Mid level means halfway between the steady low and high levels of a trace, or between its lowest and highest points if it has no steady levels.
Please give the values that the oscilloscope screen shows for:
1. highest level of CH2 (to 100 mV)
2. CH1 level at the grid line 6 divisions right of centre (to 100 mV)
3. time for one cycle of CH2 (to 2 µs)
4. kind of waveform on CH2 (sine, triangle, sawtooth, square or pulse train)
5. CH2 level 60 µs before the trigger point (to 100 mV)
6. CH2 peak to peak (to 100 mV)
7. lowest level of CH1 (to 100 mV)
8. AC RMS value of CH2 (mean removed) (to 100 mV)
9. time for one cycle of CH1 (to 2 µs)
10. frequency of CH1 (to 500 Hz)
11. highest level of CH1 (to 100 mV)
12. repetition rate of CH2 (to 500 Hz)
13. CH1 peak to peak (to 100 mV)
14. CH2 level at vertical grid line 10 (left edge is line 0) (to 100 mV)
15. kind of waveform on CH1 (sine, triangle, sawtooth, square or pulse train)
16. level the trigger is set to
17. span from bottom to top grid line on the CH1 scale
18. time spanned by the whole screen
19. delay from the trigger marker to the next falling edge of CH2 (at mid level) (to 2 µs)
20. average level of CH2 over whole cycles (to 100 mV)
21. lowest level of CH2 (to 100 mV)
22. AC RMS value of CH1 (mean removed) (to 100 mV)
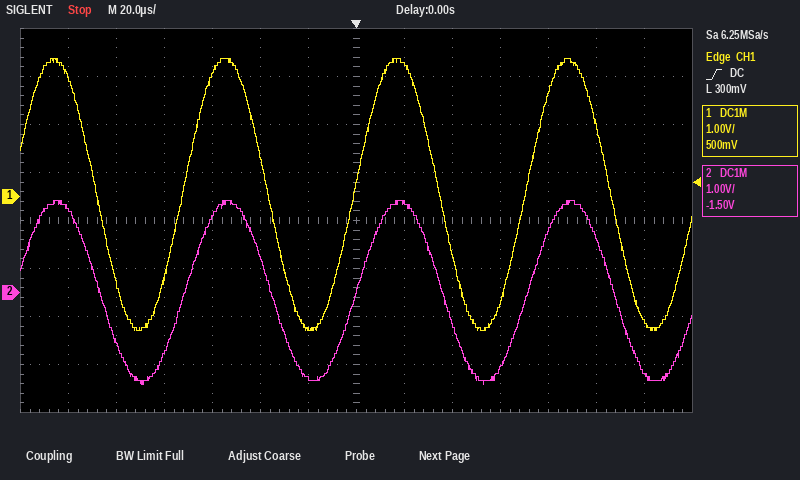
1.9 V
-2.6 V
72 µs
sine
1.6 V
3.8 V
-2.8 V
1.3 V
72 µs
14.0 kHz
2.9 V
14.0 kHz
5.7 V
-1.6 V
sine
300 mV
8 V
280 µs
36 µs
0.0 V
-1.9 V
2.0 V
